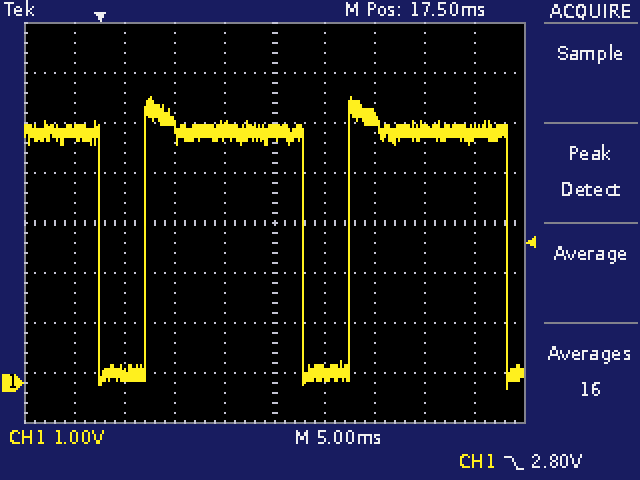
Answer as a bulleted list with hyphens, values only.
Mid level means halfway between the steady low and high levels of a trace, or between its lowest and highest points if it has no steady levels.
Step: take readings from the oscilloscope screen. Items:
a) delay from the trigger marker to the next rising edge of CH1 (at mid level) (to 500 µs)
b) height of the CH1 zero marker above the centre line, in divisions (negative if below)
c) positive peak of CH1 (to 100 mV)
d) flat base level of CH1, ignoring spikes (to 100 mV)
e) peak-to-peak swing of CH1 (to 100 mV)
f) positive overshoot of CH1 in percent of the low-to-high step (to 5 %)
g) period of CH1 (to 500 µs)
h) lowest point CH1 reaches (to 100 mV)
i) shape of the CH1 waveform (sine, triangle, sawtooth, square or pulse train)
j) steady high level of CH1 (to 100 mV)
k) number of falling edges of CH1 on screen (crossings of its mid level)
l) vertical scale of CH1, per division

- 4.5 ms
- -3.2 div
- 5.7 V
- 200 mV
- 5.8 V
- 15 %
- 20.5 ms
- -100 mV
- pulse train
- 5.0 V
- 3
- 1 V
